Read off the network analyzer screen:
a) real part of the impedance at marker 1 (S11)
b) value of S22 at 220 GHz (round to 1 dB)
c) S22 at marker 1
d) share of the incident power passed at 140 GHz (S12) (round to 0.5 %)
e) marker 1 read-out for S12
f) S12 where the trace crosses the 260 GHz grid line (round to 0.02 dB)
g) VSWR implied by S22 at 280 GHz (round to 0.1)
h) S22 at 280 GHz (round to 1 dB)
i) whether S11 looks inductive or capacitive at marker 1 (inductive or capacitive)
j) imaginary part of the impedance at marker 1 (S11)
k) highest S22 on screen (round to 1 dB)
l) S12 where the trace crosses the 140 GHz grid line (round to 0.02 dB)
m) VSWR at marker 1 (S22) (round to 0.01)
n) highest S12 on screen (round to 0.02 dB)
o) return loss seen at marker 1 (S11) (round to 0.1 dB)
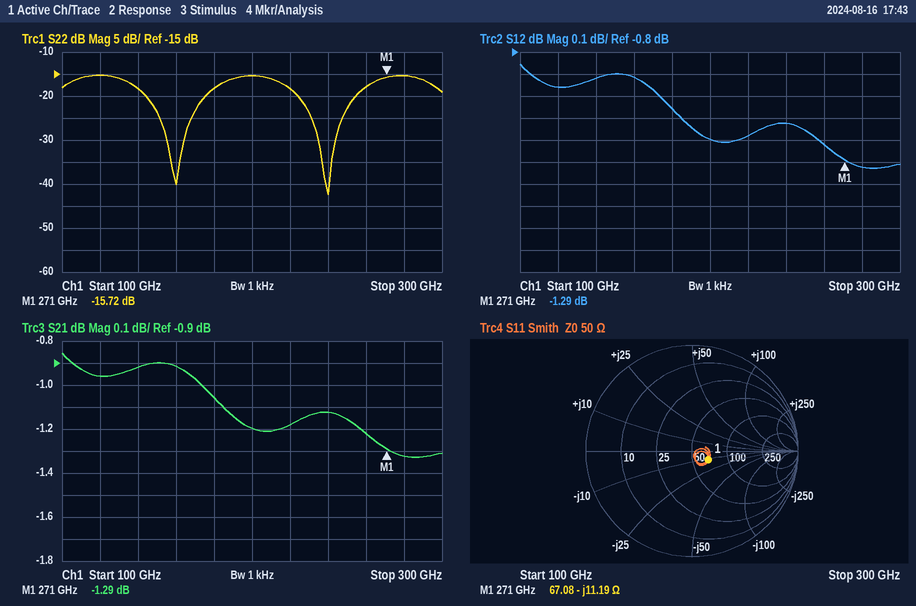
67.08 Ω
-18 dB
-15.72 dB
81.0 %
-1.29 dB
-1.22 dB
1.4
-15 dB
capacitive
-11.19 Ω
-15 dB
-0.92 dB
1.39
-0.86 dB
15.2 dB
